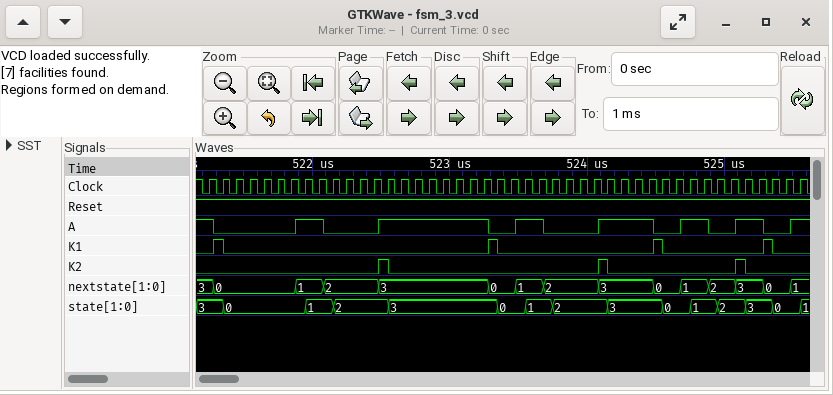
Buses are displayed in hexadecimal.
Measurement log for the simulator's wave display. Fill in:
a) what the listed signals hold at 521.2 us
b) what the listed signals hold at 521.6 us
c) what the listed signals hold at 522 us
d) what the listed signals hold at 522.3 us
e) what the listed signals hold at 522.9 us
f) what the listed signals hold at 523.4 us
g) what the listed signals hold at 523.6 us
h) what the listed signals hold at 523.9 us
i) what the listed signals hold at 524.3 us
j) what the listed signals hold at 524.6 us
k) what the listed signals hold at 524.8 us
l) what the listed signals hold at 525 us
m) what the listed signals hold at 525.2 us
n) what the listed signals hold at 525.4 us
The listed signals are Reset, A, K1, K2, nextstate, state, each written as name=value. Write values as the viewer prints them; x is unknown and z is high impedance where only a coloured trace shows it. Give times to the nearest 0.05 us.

Reset=1, A=1, K1=0, K2=0, nextstate=3, state=3
Reset=1, A=0, K1=0, K2=0, nextstate=0, state=0
Reset=1, A=1, K1=0, K2=0, nextstate=1, state=1
Reset=1, A=0, K1=0, K2=0, nextstate=2, state=2
Reset=1, A=1, K1=0, K2=0, nextstate=3, state=3
Reset=1, A=0, K1=0, K2=0, nextstate=0, state=0
Reset=1, A=1, K1=0, K2=0, nextstate=1, state=1
Reset=1, A=0, K1=0, K2=0, nextstate=2, state=2
Reset=1, A=1, K1=0, K2=0, nextstate=3, state=3
Reset=1, A=0, K1=0, K2=0, nextstate=0, state=0
Reset=1, A=1, K1=0, K2=0, nextstate=1, state=1
Reset=1, A=0, K1=0, K2=0, nextstate=2, state=2
Reset=1, A=1, K1=0, K2=0, nextstate=3, state=3
Reset=1, A=0, K1=0, K2=0, nextstate=0, state=0
